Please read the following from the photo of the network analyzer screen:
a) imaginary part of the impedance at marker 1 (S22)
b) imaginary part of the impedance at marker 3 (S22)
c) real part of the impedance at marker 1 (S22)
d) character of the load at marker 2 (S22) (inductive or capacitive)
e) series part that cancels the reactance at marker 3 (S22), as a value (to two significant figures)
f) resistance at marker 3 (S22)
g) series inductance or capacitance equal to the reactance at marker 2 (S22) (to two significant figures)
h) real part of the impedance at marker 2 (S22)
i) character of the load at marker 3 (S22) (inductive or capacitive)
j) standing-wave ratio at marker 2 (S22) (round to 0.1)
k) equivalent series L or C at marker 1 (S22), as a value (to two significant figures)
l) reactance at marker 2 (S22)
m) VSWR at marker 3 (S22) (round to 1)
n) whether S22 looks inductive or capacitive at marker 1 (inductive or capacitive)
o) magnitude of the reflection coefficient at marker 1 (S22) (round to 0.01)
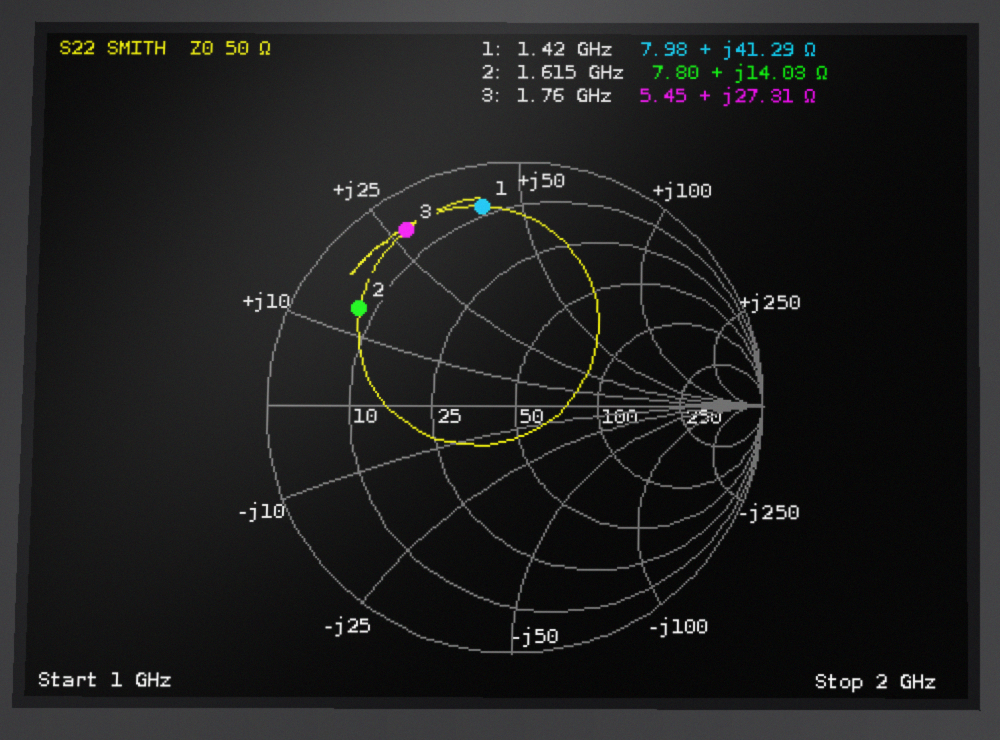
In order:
+41.29 Ω
+27.31 Ω
7.98 Ω
inductive
3.3 pF
5.45 Ω
1.4 nH
7.80 Ω
inductive
6.9
4.6 nH
+14.03 Ω
12
inductive
0.83
